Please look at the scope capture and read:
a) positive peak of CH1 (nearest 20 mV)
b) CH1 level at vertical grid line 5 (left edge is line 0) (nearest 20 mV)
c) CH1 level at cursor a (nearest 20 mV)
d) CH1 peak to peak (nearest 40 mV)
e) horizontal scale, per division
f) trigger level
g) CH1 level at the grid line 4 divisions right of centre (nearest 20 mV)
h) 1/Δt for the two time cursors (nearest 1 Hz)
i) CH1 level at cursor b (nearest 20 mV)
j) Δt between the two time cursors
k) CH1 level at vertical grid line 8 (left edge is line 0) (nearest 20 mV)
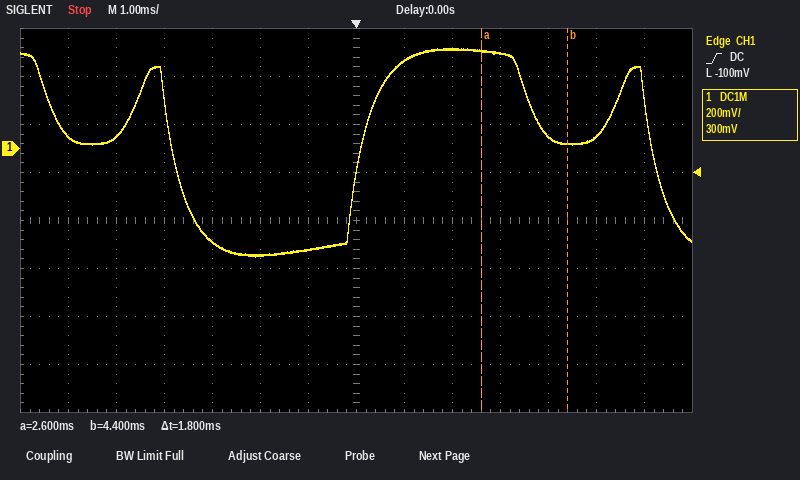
420 mV
-440 mV
400 mV
880 mV
1 ms
-100 mV
60 mV
556 Hz
20 mV
1.8 ms
360 mV
